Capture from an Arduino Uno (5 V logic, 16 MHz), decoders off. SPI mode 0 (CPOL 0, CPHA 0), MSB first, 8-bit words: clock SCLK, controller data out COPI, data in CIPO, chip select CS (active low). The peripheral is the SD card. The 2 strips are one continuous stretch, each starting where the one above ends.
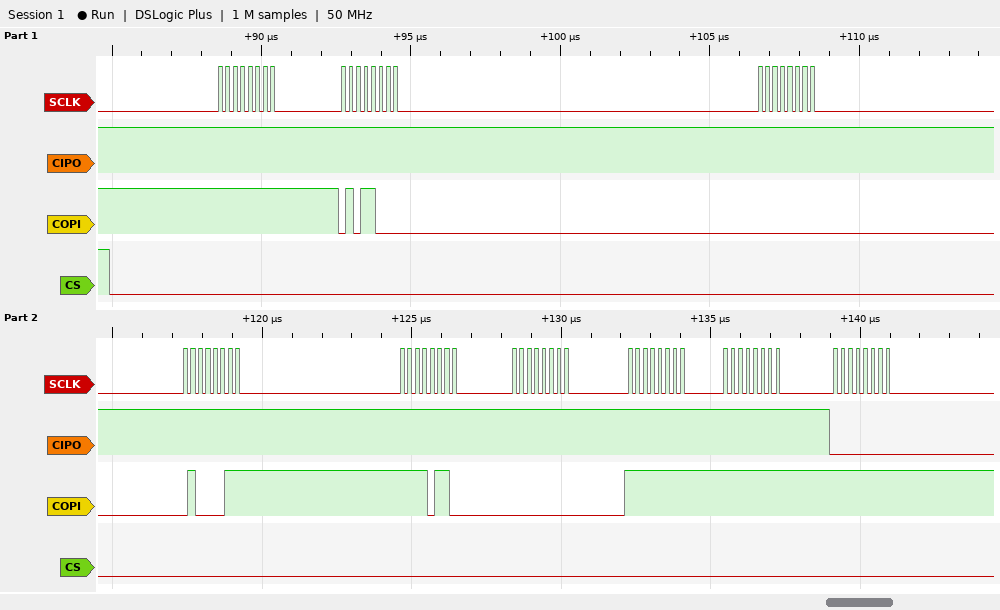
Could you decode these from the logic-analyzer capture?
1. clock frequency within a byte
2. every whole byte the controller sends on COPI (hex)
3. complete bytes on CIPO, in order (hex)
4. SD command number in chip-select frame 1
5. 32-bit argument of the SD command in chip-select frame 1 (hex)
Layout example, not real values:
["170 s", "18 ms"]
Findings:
["4 MHz", "FF 58 00 43 F6 00 FF FF FF", "FF FF FF FF FF FF FF FF 00", "CMD24", "0x0043F600"]
